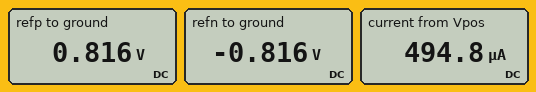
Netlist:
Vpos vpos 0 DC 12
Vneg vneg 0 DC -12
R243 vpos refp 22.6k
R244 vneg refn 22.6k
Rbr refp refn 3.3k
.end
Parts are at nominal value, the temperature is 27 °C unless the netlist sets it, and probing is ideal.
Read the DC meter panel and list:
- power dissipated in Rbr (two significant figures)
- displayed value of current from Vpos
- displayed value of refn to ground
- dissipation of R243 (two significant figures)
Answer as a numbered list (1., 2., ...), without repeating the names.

1. 810 µW
2. 494.8 µA
3. -0.816 V
4. 5.5 mW
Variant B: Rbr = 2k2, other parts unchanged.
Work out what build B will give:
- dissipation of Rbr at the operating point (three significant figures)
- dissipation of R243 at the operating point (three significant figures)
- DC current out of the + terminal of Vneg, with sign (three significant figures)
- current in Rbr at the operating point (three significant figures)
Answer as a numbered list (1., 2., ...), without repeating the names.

1. 564 µW
2. 5.79 mW
3. -506 µA
4. 506 µA
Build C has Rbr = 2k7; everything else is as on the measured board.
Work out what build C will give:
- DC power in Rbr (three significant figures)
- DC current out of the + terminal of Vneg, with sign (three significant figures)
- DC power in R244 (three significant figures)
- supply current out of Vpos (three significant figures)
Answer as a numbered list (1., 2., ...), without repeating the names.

1. 678 µW
2. -501 µA
3. 5.67 mW
4. 501 µA
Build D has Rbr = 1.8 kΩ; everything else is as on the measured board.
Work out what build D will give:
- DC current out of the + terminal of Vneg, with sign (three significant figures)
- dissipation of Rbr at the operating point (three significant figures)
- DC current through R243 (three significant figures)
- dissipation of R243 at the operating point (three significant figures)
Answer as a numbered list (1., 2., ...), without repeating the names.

1. -511 µA
2. 469 µW
3. 511 µA
4. 5.89 mW
